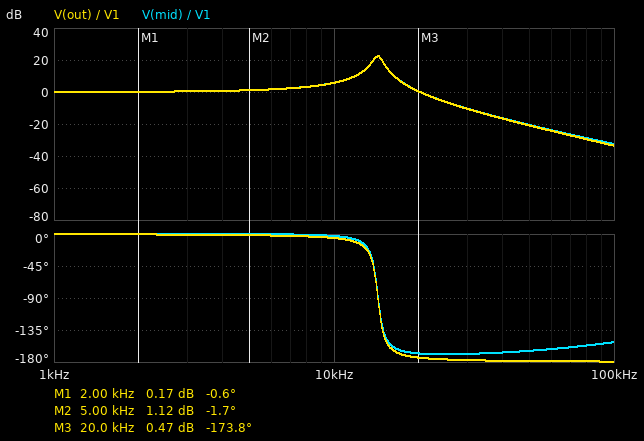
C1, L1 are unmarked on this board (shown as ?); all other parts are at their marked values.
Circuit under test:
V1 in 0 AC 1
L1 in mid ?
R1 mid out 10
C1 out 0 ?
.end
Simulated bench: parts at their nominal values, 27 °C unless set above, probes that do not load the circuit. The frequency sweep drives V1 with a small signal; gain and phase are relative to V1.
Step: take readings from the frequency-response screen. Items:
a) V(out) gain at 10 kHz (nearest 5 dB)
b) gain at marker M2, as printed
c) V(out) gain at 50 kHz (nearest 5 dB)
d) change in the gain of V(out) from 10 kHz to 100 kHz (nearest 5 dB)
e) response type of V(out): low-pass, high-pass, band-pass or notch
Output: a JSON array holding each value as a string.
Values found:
["5 dB", "1.12 dB", "-20 dB", "-40 dB", "low-pass"]
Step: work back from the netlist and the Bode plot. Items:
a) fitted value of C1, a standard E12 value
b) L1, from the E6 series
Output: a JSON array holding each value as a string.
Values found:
["82 nF", "1.5 mH"]
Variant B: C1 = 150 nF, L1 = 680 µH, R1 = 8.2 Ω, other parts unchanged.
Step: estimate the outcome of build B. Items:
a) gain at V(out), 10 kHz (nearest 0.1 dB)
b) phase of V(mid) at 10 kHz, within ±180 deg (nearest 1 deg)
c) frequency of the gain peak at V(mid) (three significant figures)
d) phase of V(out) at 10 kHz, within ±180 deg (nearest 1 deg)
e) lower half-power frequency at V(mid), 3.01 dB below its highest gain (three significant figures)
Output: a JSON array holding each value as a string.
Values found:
["4.4 dB", "-3 deg", "15.7 kHz", "-7 deg", "14.7 kHz"]
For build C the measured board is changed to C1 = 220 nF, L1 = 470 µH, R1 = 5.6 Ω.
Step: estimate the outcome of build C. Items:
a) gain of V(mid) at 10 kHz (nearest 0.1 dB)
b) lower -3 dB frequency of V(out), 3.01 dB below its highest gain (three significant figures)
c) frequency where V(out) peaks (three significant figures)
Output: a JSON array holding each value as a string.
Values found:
["4.5 dB", "14.6 kHz", "15.6 kHz"]
